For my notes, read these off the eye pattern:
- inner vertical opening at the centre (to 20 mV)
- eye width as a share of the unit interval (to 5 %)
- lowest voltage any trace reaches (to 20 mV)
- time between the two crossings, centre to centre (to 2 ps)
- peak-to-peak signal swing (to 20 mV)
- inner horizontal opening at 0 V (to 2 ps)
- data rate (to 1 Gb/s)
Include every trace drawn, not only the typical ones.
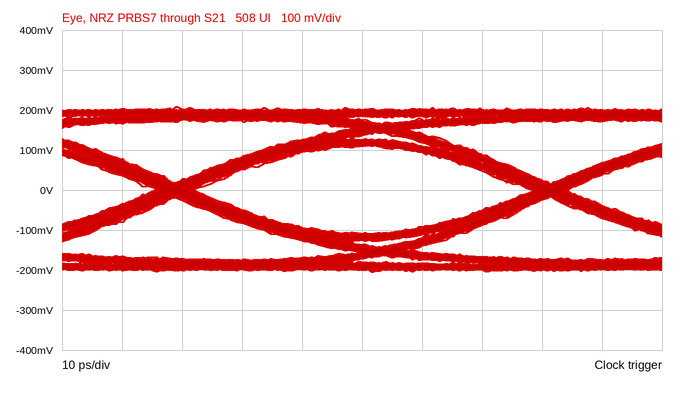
220 mV
90 %
-200 mV
62 ps
420 mV
56 ps
16 Gb/s
